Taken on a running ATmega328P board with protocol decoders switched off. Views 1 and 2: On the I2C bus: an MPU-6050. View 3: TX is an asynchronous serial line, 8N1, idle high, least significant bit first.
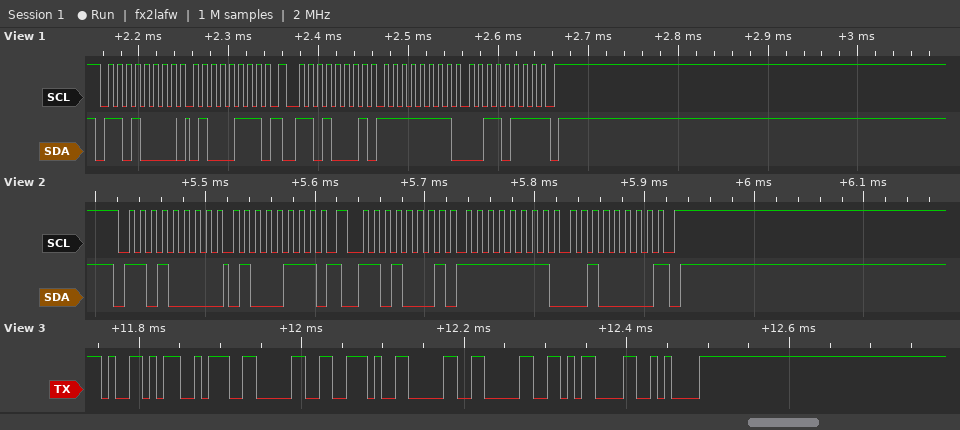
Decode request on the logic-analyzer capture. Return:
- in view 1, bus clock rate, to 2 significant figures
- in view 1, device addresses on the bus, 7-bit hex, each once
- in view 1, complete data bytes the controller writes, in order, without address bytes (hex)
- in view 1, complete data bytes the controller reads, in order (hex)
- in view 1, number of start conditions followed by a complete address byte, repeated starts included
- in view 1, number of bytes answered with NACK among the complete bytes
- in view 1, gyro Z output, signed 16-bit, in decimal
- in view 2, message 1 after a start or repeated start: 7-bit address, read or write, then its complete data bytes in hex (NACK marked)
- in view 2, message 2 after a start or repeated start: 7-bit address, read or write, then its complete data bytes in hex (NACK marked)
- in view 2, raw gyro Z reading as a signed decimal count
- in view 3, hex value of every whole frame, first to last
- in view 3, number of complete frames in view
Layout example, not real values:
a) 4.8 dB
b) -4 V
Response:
a) 100 kHz
b) 0x68
c) 47
d) FF 37
e) 2
f) 1
g) -201
h) 0x68 write: 47
i) 0x68 read: FF 20 NACK
j) -224
k) 59 3A 30 2E 30 30 0D 0A
l) 8
